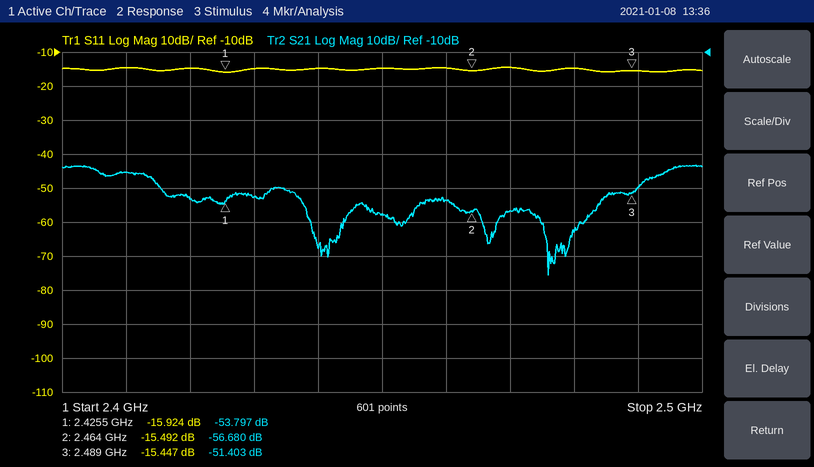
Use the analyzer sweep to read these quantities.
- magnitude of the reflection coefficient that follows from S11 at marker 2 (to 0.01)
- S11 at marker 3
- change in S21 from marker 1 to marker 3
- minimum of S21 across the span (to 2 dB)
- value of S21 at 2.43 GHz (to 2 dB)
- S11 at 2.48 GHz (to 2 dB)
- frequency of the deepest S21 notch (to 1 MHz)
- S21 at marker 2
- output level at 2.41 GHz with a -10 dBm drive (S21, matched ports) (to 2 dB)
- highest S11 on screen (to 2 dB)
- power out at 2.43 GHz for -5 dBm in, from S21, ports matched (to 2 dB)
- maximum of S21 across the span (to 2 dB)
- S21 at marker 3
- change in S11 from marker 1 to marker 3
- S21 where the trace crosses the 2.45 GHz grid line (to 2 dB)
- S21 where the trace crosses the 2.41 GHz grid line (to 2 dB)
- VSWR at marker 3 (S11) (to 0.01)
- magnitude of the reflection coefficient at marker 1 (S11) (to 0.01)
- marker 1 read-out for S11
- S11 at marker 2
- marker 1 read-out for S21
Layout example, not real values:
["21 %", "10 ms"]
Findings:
["0.17", "-15.447 dB", "2.394 dB", "-76 dB", "-52 dB", "-14 dB", "2.476 GHz", "-56.680 dB", "-56 dBm", "-14 dB", "-58 dBm", "-44 dB", "-51.403 dB", "0.477 dB", "-58 dB", "-46 dB", "1.41", "0.16", "-15.924 dB", "-15.492 dB", "-53.797 dB"]
